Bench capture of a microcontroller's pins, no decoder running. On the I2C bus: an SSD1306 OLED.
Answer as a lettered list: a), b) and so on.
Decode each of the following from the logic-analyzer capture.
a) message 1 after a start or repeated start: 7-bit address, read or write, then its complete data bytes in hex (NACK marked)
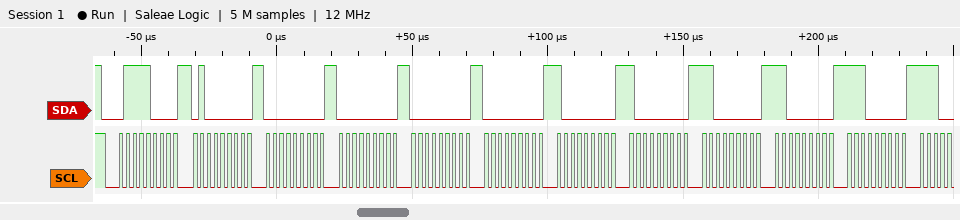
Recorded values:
a) 0x3C write: 40 00 00 00 00 80 80 C0 C0 E0
